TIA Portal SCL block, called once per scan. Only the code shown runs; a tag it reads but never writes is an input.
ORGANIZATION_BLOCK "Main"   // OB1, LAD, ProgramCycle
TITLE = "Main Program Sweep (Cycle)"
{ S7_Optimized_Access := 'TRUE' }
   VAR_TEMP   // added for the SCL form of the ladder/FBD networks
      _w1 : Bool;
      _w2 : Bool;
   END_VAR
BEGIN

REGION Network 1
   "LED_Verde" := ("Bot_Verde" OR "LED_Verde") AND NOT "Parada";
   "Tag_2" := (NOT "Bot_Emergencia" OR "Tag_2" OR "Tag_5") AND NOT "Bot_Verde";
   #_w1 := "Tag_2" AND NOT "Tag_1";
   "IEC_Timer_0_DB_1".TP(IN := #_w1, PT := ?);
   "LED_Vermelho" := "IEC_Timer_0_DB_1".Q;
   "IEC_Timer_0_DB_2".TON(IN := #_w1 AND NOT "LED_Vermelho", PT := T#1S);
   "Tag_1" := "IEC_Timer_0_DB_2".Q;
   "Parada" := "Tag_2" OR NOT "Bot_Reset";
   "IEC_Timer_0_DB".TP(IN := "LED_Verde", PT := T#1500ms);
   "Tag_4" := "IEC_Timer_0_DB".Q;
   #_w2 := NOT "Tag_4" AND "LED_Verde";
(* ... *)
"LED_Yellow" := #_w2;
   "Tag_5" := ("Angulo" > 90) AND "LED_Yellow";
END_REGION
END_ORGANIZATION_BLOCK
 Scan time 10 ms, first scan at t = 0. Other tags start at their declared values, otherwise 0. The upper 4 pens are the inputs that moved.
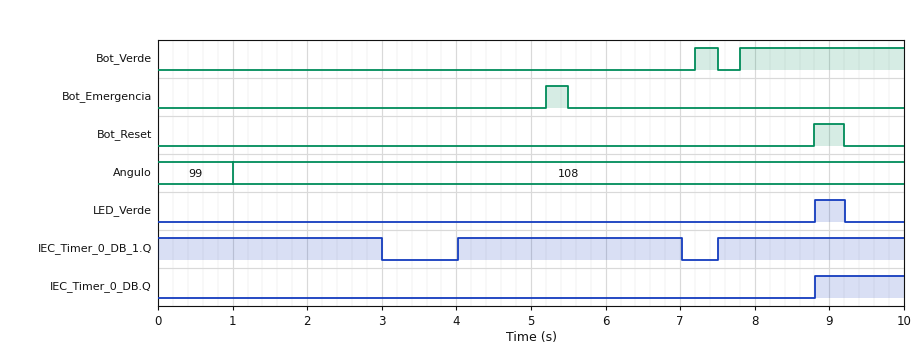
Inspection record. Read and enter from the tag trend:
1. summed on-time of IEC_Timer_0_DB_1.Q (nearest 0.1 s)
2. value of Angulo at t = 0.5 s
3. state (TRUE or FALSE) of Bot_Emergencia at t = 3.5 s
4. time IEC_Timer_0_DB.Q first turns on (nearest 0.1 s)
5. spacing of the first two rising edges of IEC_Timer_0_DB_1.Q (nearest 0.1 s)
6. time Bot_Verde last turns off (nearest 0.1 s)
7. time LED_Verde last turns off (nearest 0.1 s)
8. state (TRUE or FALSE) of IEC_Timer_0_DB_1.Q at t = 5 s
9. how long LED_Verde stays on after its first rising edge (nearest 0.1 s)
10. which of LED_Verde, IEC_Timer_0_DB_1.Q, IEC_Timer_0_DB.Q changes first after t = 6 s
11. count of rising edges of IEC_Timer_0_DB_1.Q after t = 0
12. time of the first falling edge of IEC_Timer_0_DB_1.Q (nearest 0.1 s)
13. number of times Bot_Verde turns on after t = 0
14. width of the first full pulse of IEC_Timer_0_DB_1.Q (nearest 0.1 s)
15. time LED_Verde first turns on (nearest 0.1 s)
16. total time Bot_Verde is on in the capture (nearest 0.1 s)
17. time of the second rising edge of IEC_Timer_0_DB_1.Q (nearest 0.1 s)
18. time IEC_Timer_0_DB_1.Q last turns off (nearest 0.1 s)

8.5 s
99
FALSE
8.8 s
3.5 s
7.5 s
9.2 s
TRUE
0.4 s
IEC_Timer_0_DB_1.Q
2
3.0 s
2
3.0 s
8.8 s
2.5 s
7.5 s
7.0 s
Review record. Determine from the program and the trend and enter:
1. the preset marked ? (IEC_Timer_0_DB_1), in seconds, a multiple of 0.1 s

3.0 s
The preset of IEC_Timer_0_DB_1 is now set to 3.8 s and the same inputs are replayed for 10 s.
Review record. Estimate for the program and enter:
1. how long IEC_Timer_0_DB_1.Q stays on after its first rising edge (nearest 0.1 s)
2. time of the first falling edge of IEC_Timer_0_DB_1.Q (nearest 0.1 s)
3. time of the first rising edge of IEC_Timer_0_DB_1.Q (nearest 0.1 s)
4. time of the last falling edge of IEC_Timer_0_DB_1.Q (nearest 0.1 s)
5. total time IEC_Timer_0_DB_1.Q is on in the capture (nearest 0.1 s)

3.8 s
3.8 s
4.8 s
8.6 s
7.6 s
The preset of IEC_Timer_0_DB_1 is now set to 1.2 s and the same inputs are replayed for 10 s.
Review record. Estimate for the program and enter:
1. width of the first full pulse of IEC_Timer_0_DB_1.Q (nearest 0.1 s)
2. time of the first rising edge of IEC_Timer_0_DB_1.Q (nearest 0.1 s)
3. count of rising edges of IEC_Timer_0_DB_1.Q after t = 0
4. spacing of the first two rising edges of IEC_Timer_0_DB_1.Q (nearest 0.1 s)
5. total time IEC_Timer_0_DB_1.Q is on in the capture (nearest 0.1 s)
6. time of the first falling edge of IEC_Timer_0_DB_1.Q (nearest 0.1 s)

1.2 s
2.2 s
3
2.2 s
4.8 s
1.2 s
